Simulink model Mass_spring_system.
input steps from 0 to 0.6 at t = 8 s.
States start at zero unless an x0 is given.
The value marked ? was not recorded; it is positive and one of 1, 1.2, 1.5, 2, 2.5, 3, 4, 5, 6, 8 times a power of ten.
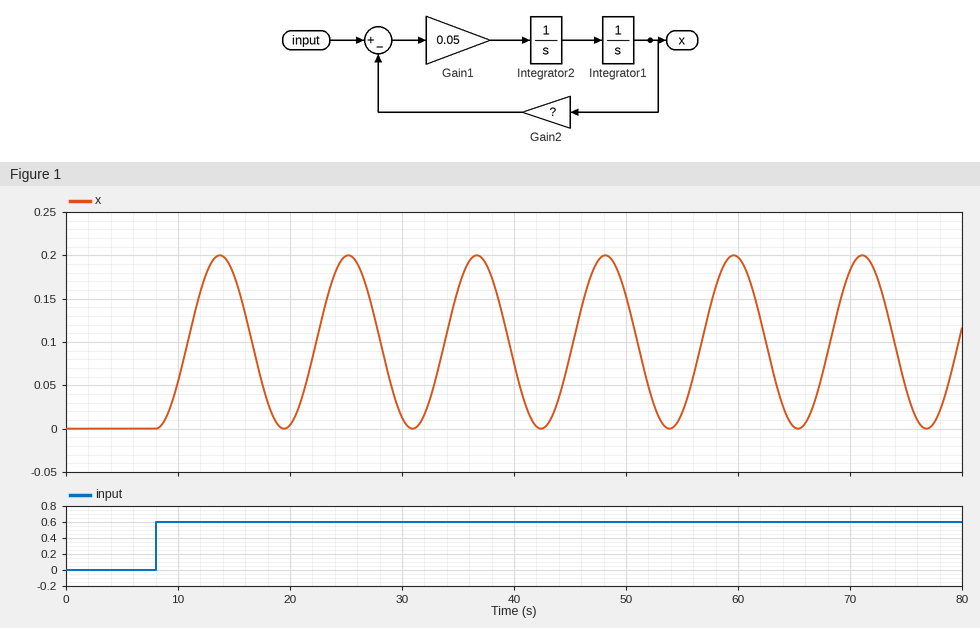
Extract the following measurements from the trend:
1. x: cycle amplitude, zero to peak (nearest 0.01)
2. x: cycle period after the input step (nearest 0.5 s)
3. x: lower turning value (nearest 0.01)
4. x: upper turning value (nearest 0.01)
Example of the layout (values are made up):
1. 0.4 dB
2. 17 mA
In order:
1. 0.10
2. 11.5 s
3. 0.00
4. 0.20
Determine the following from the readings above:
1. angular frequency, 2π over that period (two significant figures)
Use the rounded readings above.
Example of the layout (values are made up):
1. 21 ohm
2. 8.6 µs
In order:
1. 0.55 rad/s
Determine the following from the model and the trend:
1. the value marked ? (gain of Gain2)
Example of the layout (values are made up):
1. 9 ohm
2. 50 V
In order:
1. 6
